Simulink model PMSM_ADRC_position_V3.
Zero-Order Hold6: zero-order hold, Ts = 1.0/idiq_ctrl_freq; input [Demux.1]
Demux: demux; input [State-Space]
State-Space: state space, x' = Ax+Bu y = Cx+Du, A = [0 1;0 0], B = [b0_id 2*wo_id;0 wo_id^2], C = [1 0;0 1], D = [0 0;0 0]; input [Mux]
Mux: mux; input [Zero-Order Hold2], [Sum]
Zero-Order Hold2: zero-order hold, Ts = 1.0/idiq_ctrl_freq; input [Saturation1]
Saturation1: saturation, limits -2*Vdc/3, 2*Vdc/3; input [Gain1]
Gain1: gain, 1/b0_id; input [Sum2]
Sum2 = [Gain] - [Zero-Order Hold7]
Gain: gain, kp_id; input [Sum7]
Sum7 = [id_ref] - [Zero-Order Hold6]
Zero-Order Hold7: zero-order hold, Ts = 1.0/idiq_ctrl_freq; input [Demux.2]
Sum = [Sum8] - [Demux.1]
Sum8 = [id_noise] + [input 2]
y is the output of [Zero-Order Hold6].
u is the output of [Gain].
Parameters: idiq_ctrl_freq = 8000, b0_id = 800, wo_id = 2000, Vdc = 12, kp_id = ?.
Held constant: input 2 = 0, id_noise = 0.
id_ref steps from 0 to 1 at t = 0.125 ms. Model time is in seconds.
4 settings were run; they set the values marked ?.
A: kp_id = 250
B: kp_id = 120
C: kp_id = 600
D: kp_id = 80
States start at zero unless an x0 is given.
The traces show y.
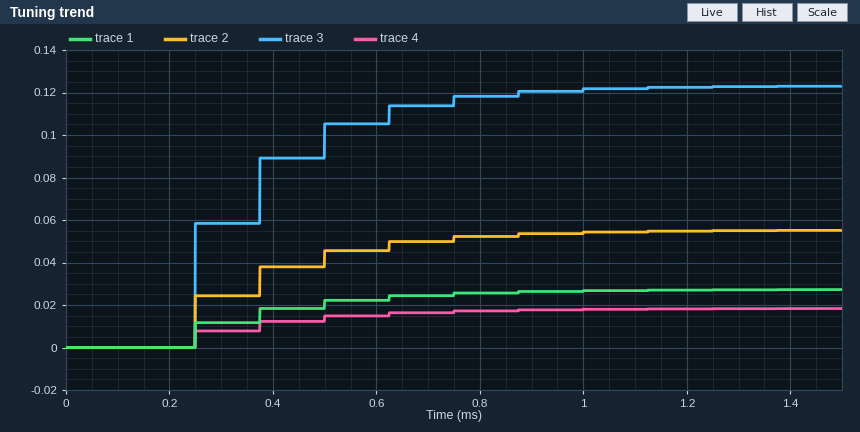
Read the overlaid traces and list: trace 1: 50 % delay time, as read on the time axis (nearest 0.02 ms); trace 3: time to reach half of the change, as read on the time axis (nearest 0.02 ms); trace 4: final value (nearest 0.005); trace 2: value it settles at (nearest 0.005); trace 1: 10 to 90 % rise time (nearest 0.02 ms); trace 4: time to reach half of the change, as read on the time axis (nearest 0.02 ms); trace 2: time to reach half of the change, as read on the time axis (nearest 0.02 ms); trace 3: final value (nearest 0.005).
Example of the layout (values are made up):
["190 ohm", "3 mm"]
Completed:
["0.38 ms", "0.38 ms", "0.020", "0.055", "0.50 ms", "0.38 ms", "0.38 ms", "0.125"]
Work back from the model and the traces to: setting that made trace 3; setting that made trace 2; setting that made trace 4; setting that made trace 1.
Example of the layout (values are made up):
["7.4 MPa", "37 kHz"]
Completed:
["C", "A", "D", "B"]
